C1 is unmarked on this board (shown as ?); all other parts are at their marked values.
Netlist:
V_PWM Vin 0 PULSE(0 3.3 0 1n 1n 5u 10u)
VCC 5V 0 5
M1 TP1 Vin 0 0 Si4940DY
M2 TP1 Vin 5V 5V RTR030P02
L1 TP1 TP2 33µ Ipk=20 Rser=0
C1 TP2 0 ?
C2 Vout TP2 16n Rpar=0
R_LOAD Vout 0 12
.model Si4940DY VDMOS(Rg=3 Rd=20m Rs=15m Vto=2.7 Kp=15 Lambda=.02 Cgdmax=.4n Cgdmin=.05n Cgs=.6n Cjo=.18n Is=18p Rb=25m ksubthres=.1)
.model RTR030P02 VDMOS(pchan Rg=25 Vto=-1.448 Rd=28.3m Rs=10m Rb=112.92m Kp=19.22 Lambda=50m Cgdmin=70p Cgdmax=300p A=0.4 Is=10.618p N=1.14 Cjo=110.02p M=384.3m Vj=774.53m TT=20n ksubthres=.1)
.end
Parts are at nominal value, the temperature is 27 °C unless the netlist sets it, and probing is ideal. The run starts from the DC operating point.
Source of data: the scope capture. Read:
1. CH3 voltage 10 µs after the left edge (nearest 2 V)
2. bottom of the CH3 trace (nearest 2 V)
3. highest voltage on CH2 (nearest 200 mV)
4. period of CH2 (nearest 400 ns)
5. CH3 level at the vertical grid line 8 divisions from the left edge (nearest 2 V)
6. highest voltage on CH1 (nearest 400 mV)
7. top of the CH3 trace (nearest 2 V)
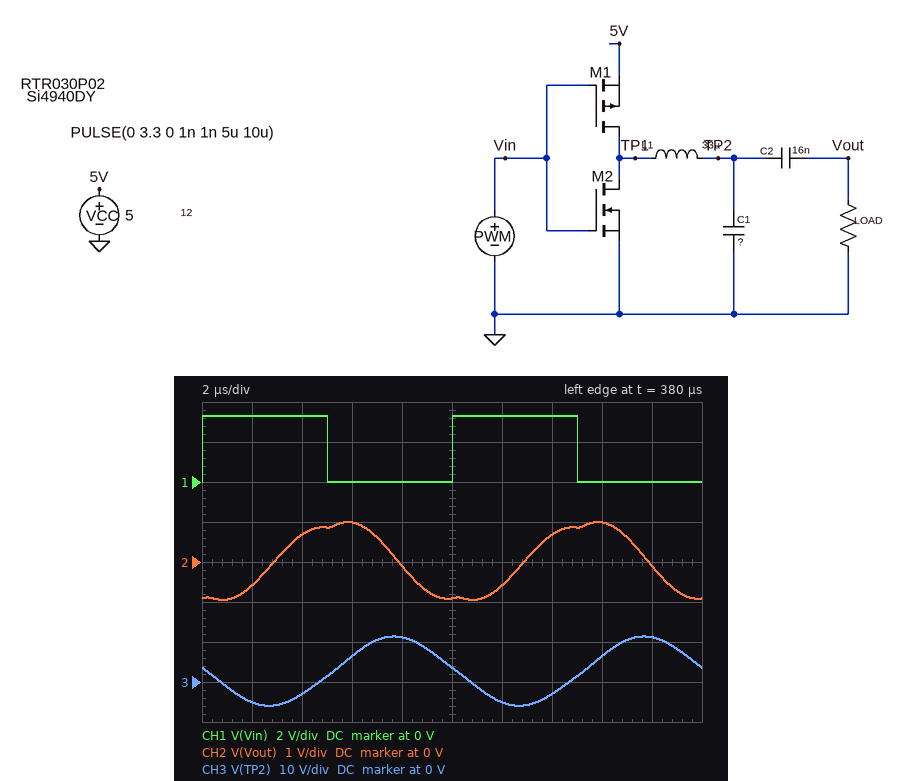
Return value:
4 V
-6 V
1.0 V
10.0 µs
6 V
3.2 V
12 V
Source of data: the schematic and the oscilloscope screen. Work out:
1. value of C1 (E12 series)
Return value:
33 nF
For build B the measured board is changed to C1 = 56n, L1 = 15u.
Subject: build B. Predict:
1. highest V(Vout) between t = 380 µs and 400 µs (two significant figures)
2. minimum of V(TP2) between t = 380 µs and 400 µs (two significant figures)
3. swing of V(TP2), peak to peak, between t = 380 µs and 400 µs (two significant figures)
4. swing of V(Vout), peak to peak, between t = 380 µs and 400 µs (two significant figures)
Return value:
670 mV
-2.9 V
11 V
1.3 V
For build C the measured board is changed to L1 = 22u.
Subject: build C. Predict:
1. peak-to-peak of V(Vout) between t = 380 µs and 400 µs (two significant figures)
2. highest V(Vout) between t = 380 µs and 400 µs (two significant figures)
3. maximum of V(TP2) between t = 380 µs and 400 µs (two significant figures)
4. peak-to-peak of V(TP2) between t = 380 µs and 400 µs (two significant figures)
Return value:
1.3 V
680 mV
8.5 V
11 V
